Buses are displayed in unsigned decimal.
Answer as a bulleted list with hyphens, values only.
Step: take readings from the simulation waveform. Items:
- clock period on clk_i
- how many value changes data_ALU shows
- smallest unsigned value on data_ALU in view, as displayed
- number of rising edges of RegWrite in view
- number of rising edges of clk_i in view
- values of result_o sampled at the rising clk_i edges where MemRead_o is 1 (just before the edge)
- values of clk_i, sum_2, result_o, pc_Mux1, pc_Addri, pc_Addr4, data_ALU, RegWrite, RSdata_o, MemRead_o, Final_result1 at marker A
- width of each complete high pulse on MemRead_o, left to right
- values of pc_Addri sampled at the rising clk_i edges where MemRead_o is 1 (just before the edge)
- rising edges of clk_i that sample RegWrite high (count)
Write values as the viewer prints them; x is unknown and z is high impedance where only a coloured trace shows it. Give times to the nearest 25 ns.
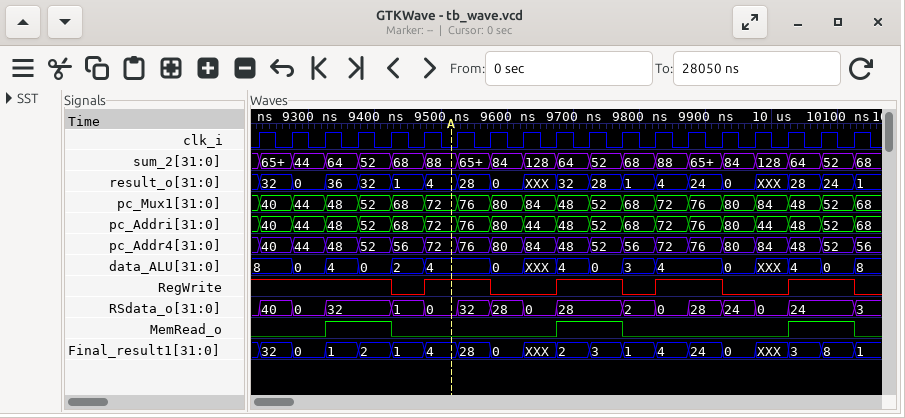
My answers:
- 50 ns
- 16
- 0
- 4
- 19
- 36, 32, 32, 28, 28, 24
- clk_i=0, sum_2=88, result_o=4, pc_Mux1=72, pc_Addri=72, pc_Addr4=72, data_ALU=4, RegWrite=1, RSdata_o=0, MemRead_o=0, Final_result1=4
- 100 ns, 100 ns, 100 ns
- 48, 52, 48, 52, 48, 52
- 13
